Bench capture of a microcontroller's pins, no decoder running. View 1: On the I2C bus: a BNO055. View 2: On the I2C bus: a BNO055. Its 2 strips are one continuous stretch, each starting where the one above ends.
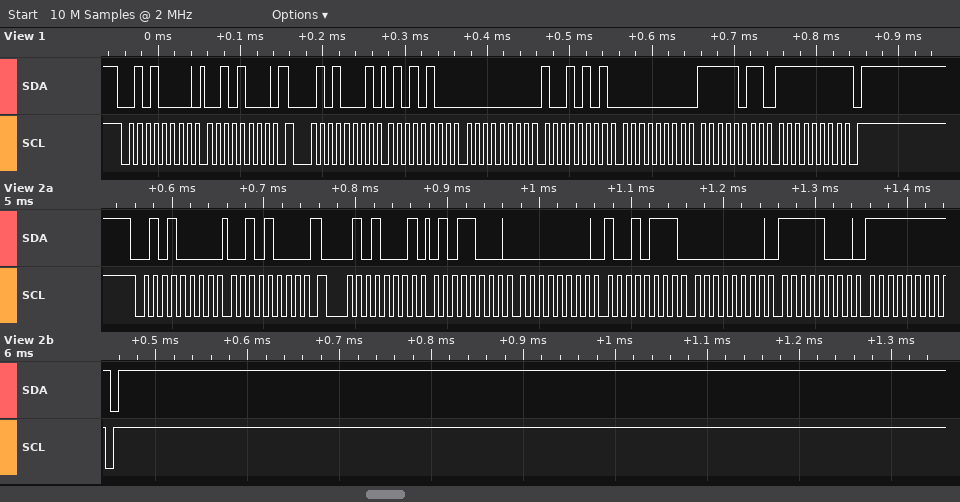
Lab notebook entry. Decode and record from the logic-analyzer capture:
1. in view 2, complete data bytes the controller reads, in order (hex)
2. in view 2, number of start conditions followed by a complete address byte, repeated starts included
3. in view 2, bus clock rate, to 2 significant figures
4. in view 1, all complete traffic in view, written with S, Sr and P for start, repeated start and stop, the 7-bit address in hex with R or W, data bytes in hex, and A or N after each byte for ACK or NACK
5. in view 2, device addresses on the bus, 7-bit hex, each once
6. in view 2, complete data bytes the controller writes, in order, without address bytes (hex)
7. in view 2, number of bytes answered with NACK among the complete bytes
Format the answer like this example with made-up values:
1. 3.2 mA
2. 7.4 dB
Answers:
1. 58 00 97 00 F8 FF
2. 2
3. 100 kHz
4. S 28W A 28 A Sr 28R A 54 A 00 A 95 A 00 A FB A FF N P
5. 0x28
6. 28
7. 1
